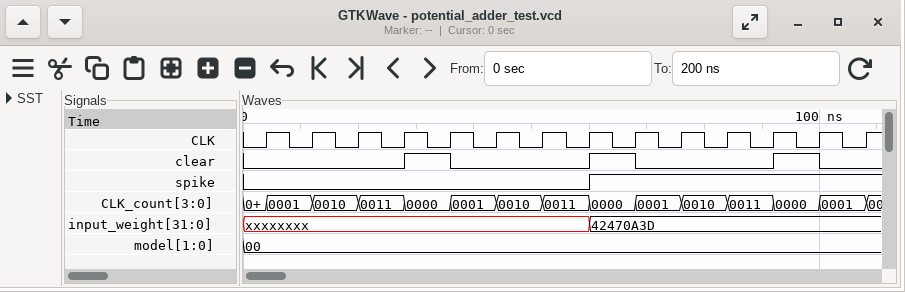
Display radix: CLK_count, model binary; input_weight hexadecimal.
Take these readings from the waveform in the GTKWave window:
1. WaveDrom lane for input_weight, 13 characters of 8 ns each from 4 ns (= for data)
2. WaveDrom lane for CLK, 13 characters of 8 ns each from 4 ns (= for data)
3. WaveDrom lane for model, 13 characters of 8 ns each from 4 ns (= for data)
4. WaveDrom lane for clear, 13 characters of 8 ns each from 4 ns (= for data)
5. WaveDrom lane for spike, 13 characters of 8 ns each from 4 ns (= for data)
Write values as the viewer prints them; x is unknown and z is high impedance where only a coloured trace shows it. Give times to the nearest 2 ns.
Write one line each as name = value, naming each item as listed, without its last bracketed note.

WaveDrom lane for input_weight, 13 characters of 8 ns each from 4 ns = {name: 'input_weight', wave: 'x......=.....', data: '42470A3D'}
WaveDrom lane for CLK, 13 characters of 8 ns each from 4 ns = {name: 'CLK', wave: 'p............'}
WaveDrom lane for model, 13 characters of 8 ns each from 4 ns = {name: 'model', wave: '=............', data: '00'}
WaveDrom lane for clear, 13 characters of 8 ns each from 4 ns = {name: 'clear', wave: '0..10..10..10'}
WaveDrom lane for spike, 13 characters of 8 ns each from 4 ns = {name: 'spike', wave: '0......1.....'}
